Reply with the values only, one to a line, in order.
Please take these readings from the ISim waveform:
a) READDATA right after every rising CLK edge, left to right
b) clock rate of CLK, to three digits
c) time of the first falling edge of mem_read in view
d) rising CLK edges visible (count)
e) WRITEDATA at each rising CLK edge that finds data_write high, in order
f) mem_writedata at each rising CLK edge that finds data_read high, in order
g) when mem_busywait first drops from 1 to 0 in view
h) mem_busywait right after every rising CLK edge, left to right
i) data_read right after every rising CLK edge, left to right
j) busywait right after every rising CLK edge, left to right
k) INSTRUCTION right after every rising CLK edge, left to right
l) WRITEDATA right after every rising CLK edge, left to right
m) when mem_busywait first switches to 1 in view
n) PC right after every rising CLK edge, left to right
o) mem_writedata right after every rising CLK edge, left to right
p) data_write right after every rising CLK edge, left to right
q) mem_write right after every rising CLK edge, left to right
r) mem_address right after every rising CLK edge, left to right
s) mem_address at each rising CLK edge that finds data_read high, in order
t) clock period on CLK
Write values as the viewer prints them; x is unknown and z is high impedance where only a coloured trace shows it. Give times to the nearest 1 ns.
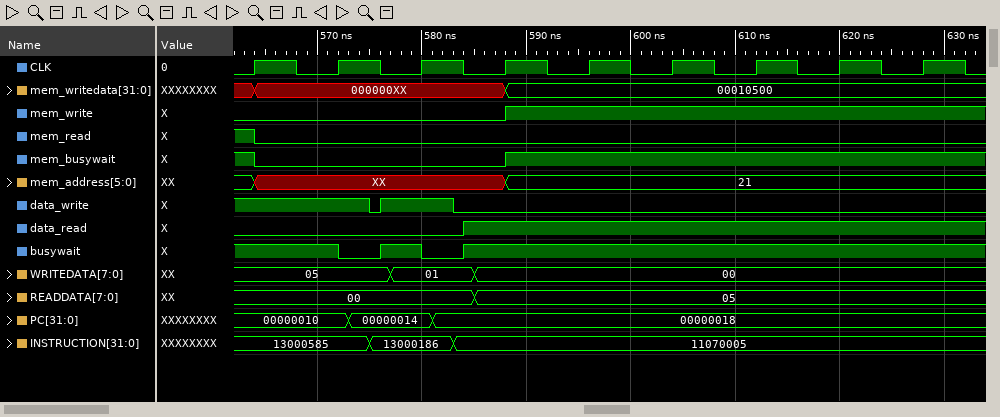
00, 00, 00, 05, 05, 05, 05, 05, 05
125 MHz
564 ns
9
05, 05, 01
000000XX, 00010500, 00010500, 00010500, 00010500, 00010500
564 ns
0 0 0 1 1 1 1 1 1
0 0 0 1 1 1 1 1 1
1 0 0 1 1 1 1 1 1
13000585, 13000585, 13000186, 11070005, 11070005, 11070005, 11070005, 11070005, 11070005
05, 05, 01, 00, 00, 00, 00, 00, 00
588 ns
00000010, 00000010, 00000014, 00000018, 00000018, 00000018, 00000018, 00000018, 00000018
000000XX, 000000XX, 000000XX, 00010500, 00010500, 00010500, 00010500, 00010500, 00010500
1 1 1 0 0 0 0 0 0
0 0 0 1 1 1 1 1 1
XX, XX, XX, 21, 21, 21, 21, 21, 21
XX, 21, 21, 21, 21, 21
8 ns
